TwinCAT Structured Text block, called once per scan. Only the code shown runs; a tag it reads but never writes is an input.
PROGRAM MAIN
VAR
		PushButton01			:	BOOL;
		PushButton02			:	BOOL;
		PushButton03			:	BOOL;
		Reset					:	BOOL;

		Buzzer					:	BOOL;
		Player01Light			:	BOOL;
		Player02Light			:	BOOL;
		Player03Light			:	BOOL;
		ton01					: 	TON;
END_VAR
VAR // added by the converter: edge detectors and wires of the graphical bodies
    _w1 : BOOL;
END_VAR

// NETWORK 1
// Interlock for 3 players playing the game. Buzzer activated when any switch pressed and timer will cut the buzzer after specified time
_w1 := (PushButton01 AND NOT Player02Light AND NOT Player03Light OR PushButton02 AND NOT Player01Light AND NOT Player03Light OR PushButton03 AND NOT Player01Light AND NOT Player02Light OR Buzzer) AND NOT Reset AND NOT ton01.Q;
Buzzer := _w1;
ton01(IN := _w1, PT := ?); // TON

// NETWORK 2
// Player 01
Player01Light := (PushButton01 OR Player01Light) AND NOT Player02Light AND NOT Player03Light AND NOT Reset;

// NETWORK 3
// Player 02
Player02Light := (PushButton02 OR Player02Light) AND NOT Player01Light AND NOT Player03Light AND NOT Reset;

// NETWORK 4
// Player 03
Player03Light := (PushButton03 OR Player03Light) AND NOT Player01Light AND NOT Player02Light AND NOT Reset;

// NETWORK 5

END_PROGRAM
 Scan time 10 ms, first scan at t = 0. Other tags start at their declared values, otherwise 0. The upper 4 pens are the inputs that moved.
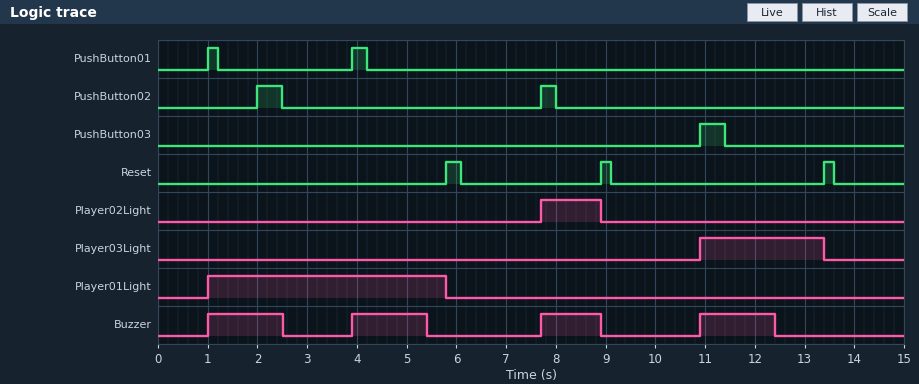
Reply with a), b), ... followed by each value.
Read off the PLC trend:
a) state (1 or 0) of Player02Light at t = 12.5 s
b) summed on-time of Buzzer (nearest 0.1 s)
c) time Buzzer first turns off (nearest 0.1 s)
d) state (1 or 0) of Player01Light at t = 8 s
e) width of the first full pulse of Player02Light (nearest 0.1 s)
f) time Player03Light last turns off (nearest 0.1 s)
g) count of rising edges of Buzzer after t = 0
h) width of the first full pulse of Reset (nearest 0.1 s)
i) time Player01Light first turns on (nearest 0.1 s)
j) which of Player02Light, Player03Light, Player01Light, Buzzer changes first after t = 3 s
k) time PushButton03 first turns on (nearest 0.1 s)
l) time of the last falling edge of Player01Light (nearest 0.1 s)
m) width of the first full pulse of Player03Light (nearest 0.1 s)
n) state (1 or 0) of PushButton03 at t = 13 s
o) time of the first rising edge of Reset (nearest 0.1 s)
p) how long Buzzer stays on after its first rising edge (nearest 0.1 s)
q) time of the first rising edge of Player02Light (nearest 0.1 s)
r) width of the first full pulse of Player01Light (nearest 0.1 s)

a) 0
b) 5.7 s
c) 2.5 s
d) 0
e) 1.2 s
f) 13.4 s
g) 4
h) 0.3 s
i) 1.0 s
j) Buzzer
k) 10.9 s
l) 5.8 s
m) 2.5 s
n) 0
o) 5.8 s
p) 1.5 s
q) 7.7 s
r) 4.8 s
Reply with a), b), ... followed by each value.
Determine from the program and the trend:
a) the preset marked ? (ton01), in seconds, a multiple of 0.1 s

a) 1.5 s
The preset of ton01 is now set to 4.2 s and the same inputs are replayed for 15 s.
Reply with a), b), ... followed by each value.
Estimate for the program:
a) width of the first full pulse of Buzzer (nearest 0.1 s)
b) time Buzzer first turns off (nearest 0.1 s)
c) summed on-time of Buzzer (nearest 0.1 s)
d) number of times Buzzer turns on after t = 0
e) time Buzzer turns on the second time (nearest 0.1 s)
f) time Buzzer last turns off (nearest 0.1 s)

a) 4.2 s
b) 5.2 s
c) 7.9 s
d) 3
e) 7.7 s
f) 13.4 s
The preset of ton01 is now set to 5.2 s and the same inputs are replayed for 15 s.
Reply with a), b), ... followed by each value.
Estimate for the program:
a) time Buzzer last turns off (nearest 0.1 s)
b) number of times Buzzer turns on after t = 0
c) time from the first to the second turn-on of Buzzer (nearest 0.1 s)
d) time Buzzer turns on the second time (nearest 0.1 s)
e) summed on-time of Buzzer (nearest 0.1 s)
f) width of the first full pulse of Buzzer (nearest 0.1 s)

a) 13.4 s
b) 3
c) 6.7 s
d) 7.7 s
e) 8.5 s
f) 4.8 s
